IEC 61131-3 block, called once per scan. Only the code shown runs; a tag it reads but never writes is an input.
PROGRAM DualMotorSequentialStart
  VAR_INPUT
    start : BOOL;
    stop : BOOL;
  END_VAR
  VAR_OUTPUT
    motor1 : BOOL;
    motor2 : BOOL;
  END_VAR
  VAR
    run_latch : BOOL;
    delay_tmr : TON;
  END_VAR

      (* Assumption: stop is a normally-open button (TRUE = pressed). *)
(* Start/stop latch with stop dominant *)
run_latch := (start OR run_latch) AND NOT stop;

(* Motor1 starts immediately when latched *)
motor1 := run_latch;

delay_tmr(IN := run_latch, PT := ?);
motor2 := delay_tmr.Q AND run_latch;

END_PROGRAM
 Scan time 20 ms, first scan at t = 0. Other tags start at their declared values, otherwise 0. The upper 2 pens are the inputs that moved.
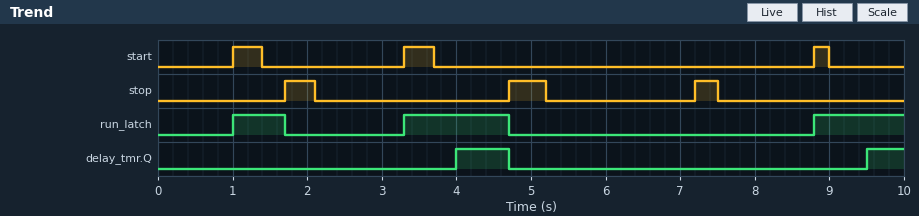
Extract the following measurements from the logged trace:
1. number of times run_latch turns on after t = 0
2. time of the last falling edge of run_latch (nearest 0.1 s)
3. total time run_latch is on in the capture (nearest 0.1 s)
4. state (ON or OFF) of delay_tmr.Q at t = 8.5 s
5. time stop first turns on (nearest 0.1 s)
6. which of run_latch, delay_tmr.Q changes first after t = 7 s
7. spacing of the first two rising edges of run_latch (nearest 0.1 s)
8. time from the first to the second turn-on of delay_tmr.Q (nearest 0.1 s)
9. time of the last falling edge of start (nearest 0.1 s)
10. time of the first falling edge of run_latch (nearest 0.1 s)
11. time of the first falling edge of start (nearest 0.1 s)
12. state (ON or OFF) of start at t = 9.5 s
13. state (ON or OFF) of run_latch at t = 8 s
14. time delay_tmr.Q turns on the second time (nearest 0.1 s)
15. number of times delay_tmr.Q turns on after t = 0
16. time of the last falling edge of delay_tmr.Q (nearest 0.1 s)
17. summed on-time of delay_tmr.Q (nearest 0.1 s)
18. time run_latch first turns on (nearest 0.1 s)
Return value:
3
4.7 s
3.3 s
OFF
1.7 s
run_latch
2.3 s
5.5 s
9.0 s
1.7 s
1.4 s
OFF
OFF
9.5 s
2
4.7 s
1.2 s
1.0 s
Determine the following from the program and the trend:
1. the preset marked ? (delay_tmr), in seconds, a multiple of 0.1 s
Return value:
0.7 s
